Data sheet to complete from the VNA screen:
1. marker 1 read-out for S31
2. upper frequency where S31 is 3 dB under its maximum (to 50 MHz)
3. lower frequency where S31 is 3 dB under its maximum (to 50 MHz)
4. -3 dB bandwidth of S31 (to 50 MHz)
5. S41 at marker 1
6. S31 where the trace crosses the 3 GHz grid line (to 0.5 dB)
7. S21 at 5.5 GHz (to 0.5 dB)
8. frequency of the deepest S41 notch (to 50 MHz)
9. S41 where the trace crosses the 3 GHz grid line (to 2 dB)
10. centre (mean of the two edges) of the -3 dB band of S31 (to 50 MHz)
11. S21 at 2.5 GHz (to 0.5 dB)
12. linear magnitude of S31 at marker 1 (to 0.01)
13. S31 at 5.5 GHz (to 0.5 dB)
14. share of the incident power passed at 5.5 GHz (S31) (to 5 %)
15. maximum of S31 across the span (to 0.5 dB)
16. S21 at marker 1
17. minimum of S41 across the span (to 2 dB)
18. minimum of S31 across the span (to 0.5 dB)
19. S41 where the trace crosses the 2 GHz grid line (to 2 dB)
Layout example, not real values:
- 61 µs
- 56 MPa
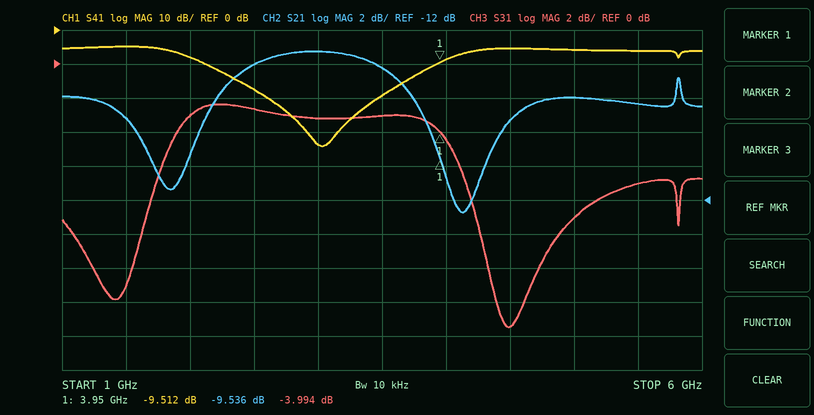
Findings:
- -3.994 dB
- 4.05 GHz
- 1.80 GHz
- 2.25 GHz
- -9.512 dB
- -3.0 dB
- -6.5 dB
- 3.05 GHz
- -34 dB
- 2.95 GHz
- -4.0 dB
- 0.63
- -7.0 dB
- 20 %
- -2.5 dB
- -9.536 dB
- -34 dB
- -15.5 dB
- -8 dB
